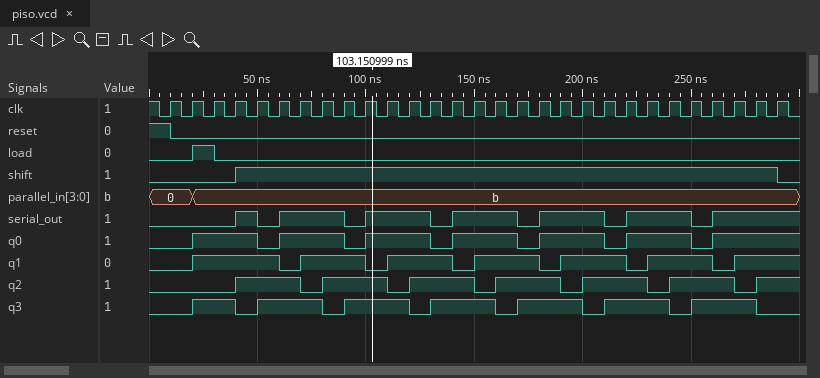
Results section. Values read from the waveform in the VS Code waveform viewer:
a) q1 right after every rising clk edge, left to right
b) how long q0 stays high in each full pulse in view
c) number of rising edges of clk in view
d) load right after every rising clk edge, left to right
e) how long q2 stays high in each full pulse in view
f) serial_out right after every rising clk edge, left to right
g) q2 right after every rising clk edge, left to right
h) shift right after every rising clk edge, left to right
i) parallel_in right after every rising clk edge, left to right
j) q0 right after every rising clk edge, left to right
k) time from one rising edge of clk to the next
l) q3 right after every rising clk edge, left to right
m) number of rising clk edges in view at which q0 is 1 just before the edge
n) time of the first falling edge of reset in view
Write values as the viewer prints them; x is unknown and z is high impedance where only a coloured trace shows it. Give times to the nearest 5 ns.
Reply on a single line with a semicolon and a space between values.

0 1 1 1 1 0 1 1 1 0 1 1 1 0 1 1 1 0 1 1 1 0 1 1 1 0 1 1 1; 30 ns, 30 ns, 30 ns, 30 ns, 30 ns, 30 ns; 29; 0 1 0 0 0 0 0 0 0 0 0 0 0 0 0 0 0 0 0 0 0 0 0 0 0 0 0 0 0; 30 ns, 30 ns, 30 ns, 30 ns, 30 ns, 30 ns; 0 0 0 1 0 1 1 1 0 1 1 1 0 1 1 1 0 1 1 1 0 1 1 1 0 1 1 1 1; 0 0 0 1 1 1 0 1 1 1 0 1 1 1 0 1 1 1 0 1 1 1 0 1 1 1 0 1 1; 0 0 0 1 1 1 1 1 1 1 1 1 1 1 1 1 1 1 1 1 1 1 1 1 1 1 1 1 0; 0, b, b, b, b, b, b, b, b, b, b, b, b, b, b, b, b, b, b, b, b, b, b, b, b, b, b, b, b; 0 1 1 1 0 1 1 1 0 1 1 1 0 1 1 1 0 1 1 1 0 1 1 1 0 1 1 1 1; 10 ns; 0 1 1 0 1 1 1 0 1 1 1 0 1 1 1 0 1 1 1 0 1 1 1 0 1 1 1 0 0; 21; 10 ns
